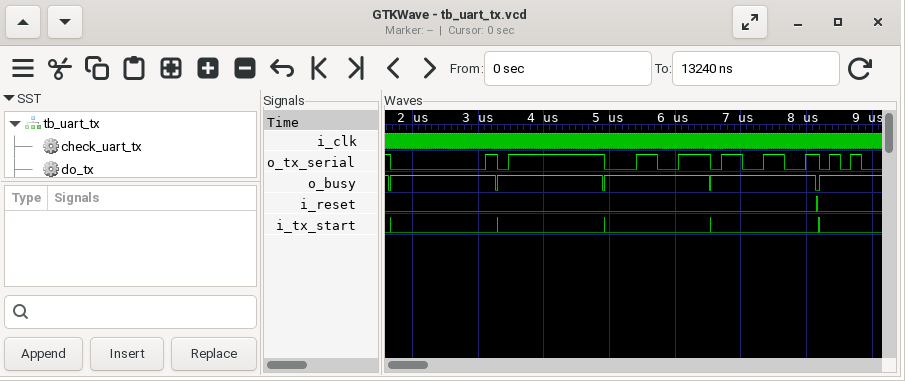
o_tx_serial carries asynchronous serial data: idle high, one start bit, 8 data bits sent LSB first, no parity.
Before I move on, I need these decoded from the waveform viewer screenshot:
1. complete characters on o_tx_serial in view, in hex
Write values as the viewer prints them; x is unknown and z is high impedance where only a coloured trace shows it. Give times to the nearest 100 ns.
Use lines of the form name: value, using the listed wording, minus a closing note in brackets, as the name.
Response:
complete characters on o_tx_serial in view, in hex: 00, FF, CC, 33
